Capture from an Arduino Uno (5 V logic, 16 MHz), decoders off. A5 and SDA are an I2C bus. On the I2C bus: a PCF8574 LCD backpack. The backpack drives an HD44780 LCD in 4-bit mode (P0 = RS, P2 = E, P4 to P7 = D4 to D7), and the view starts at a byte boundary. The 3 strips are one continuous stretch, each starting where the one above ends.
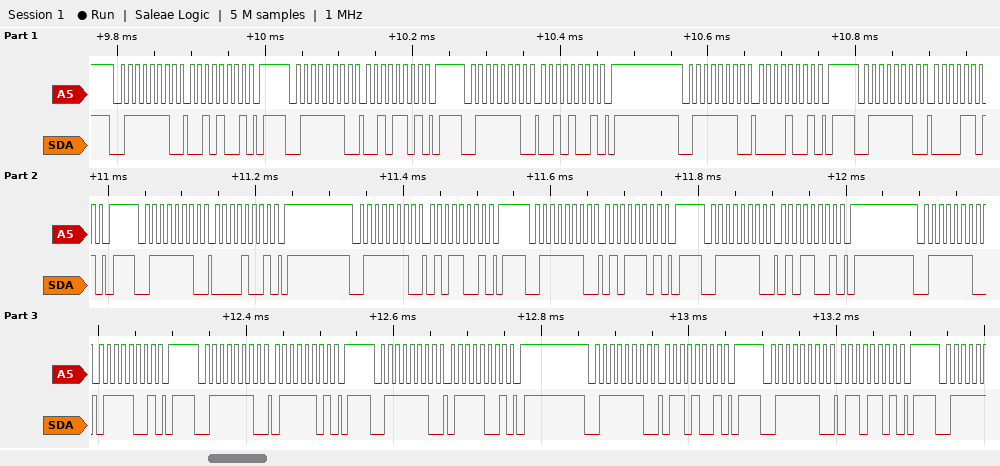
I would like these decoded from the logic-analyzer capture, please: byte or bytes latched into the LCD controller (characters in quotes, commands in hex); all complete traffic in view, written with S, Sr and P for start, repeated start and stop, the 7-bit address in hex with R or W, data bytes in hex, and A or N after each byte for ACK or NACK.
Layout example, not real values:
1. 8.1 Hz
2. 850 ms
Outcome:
1. ' ' 'W'
2. S 3FW A 29 A P S 3FW A 2D A P S 3FW A 29 A P S 3FW A 09 A P S 3FW A 0D A P S 3FW A 09 A P S 3FW A 59 A P S 3FW A 5D A P S 3FW A 59 A P S 3FW A 79 A P S 3FW A 7D A P S 3FW A 79 A P S 3FW A 69 A P S 3FW A 6D A P
